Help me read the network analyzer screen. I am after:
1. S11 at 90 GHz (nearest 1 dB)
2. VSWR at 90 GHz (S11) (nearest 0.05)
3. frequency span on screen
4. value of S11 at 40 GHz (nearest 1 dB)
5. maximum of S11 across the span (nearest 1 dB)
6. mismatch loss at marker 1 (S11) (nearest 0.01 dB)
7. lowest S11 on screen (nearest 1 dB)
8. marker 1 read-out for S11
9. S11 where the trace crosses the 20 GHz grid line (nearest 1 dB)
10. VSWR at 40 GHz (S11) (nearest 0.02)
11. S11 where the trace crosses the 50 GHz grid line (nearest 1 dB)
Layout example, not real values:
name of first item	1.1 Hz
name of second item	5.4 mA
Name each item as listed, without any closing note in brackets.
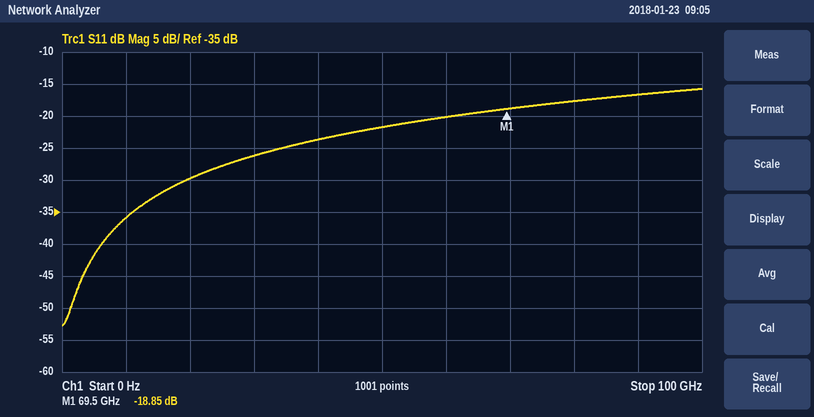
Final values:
S11 at 90 GHz	-17 dB
VSWR at 90 GHz (S11)	1.35
frequency span on screen	100 GHz
value of S11 at 40 GHz	-24 dB
maximum of S11 across the span	-16 dB
mismatch loss at marker 1 (S11)	0.06 dB
lowest S11 on screen	-53 dB
marker 1 read-out for S11	-18.85 dB
S11 where the trace crosses the 20 GHz grid line	-30 dB
VSWR at 40 GHz (S11)	1.14
S11 where the trace crosses the 50 GHz grid line	-22 dB
